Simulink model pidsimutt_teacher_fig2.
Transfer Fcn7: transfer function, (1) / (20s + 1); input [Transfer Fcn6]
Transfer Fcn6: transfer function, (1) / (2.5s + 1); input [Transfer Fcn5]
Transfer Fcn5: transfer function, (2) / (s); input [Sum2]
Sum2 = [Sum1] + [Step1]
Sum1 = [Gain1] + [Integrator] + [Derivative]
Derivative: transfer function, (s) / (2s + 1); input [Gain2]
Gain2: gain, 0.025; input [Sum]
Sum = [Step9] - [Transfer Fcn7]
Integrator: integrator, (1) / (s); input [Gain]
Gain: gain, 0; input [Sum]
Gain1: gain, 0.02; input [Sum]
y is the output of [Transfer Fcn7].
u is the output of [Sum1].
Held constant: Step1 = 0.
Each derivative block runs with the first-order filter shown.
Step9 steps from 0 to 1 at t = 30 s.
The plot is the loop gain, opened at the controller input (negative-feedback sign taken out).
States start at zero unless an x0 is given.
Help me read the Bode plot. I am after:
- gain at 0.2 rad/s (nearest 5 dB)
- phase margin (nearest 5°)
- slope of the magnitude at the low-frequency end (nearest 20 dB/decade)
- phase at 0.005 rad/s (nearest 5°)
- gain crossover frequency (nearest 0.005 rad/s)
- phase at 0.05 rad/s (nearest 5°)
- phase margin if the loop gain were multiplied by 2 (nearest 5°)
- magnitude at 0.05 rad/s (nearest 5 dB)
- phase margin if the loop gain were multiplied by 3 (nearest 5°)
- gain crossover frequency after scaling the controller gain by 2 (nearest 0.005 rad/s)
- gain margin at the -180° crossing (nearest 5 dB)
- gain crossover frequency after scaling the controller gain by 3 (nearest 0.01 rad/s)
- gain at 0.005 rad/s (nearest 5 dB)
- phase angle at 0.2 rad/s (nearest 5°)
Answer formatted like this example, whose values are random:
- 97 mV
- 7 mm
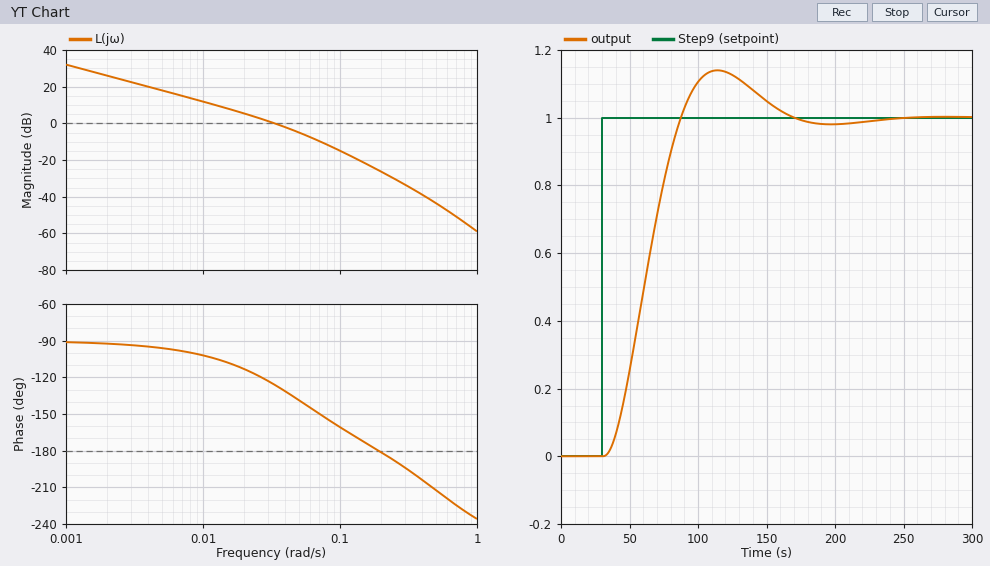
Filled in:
- -25 dB
- 55°
- -20 dB/decade
- -95°
- 0.035 rad/s
- -140°
- 40°
- -5 dB
- 30°
- 0.055 rad/s
- 25 dB
- 0.07 rad/s
- 20 dB
- -180°
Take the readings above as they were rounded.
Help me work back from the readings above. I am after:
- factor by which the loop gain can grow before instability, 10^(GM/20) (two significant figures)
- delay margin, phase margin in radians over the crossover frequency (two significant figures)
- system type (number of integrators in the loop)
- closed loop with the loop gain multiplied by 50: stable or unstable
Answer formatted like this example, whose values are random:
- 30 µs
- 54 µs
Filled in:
- 18
- 27 s
- 1
- unstable
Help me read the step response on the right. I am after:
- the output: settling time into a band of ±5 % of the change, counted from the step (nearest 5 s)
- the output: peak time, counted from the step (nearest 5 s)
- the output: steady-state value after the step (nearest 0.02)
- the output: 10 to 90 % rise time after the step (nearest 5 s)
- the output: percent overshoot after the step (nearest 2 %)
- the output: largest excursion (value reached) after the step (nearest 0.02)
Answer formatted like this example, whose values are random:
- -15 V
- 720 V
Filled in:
- 120 s
- 85 s
- 1.00
- 40 s
- 14 %
- 1.14
